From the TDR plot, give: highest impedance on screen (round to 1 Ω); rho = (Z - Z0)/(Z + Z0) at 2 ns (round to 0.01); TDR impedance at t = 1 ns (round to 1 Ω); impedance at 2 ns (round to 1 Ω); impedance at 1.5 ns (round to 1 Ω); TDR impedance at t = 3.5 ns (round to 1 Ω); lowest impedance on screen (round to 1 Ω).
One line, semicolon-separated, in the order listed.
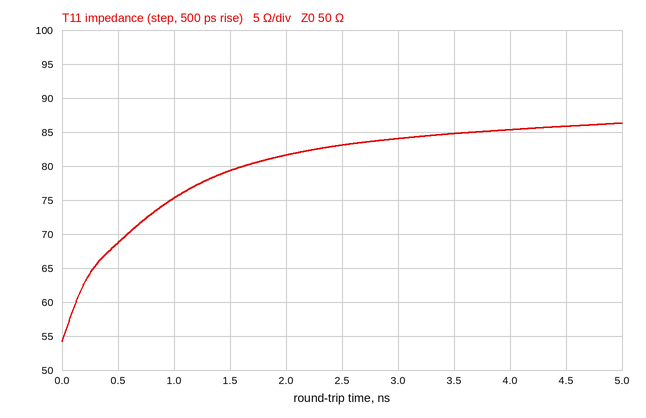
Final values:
86 Ω; +0.24; 75 Ω; 82 Ω; 79 Ω; 85 Ω; 54 Ω
